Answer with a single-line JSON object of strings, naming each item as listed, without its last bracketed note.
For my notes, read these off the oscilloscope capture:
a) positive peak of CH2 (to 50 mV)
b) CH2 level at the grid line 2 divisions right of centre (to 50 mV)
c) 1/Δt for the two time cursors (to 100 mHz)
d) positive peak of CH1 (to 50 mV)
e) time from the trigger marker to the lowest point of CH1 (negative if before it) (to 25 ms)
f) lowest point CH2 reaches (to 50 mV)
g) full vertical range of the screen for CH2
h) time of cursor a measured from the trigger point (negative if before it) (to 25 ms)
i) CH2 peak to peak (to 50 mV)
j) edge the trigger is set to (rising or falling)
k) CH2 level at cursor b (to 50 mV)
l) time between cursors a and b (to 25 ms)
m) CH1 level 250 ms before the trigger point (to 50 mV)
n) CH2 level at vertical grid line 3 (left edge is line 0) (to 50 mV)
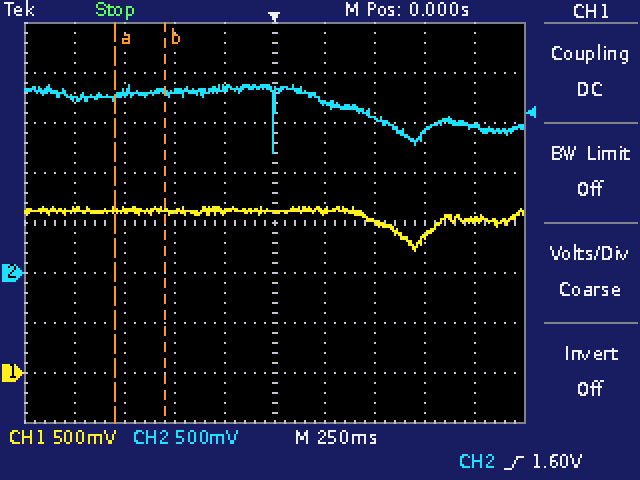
{"positive peak of CH2": "1.90 V", "CH2 level at the grid line 2 divisions right of centre": "1.55 V", "1/Δt for the two time cursors": "4.0 Hz", "positive peak of CH1": "1.65 V", "time from the trigger marker to the lowest point of CH1 (negative if before it)": "+700 ms", "lowest point CH2 reaches": "1.20 V", "full vertical range of the screen for CH2": "4 V", "time of cursor a measured from the trigger point (negative if before it)": "-800 ms", "CH2 peak to peak": "700 mV", "edge the trigger is set to": "rising", "CH2 level at cursor b": "1.80 V", "time between cursors a and b": "250 ms", "CH1 level 250 ms before the trigger point": "1.60 V", "CH2 level at vertical grid line 3 (left edge is line 0)": "1.80 V"}
